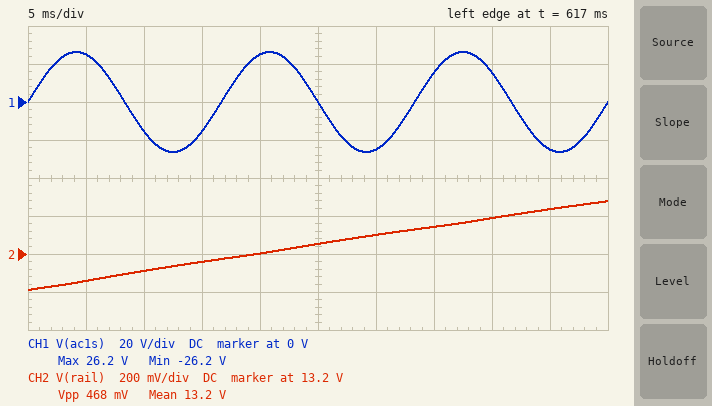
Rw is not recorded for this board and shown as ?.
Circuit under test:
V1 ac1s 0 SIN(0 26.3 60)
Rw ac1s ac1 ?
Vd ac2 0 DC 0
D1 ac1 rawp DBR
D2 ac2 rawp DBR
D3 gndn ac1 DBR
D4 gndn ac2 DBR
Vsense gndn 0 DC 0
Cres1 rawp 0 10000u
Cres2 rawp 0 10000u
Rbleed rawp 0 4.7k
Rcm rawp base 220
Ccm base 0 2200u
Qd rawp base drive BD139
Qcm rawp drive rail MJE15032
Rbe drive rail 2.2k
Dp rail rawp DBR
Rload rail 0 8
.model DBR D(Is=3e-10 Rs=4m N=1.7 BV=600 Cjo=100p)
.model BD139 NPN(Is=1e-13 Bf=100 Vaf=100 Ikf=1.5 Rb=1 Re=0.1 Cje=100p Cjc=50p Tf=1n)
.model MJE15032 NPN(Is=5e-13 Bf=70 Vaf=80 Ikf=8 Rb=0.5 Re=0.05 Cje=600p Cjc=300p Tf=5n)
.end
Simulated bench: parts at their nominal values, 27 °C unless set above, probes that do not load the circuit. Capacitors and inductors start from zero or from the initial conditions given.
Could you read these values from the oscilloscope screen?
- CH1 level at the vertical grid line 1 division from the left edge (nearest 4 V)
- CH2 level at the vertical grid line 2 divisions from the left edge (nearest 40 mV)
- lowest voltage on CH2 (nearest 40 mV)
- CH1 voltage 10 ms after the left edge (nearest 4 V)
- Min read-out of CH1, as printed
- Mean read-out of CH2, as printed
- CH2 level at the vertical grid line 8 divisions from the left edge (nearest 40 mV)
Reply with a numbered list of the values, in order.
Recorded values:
1. 24 V
2. 13.12 V
3. 13.00 V
4. -16 V
5. -26.2 V
6. 13.2 V
7. 13.40 V
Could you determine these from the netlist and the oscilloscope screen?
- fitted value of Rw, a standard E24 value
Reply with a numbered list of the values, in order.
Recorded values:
1. 0.51 Ω
